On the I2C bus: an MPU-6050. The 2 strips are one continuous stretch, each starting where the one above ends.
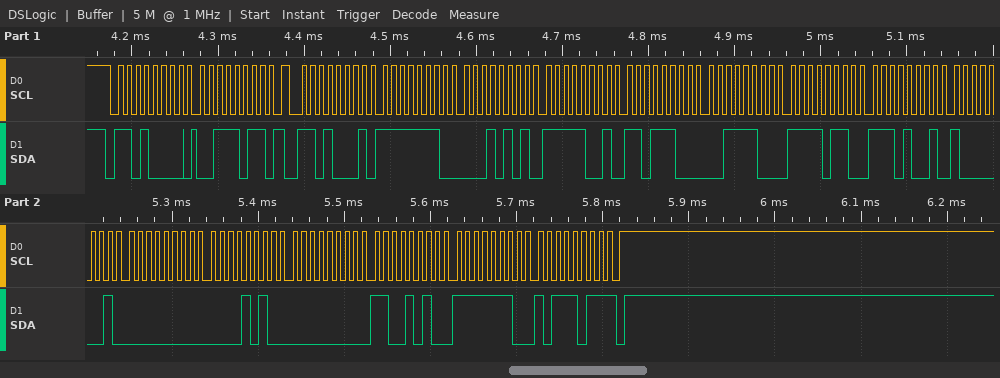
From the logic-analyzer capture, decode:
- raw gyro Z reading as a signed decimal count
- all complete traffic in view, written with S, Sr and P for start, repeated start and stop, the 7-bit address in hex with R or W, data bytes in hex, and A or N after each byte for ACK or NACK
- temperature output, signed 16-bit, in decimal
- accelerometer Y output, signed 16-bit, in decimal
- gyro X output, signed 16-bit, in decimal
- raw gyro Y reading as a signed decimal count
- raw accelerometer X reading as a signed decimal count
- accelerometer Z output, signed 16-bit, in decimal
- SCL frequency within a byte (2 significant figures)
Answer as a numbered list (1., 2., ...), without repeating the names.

1. -325
2. S 68W A 3B A Sr 68R A FE A 15 A F9 A DC A 3C A F6 A E9 A 81 A 00 A 0A A 00 A CA A FE A BB N P
3. -5759
4. -1572
5. 10
6. 202
7. -491
8. 15606
9. 100 kHz
